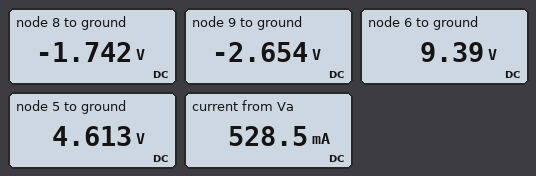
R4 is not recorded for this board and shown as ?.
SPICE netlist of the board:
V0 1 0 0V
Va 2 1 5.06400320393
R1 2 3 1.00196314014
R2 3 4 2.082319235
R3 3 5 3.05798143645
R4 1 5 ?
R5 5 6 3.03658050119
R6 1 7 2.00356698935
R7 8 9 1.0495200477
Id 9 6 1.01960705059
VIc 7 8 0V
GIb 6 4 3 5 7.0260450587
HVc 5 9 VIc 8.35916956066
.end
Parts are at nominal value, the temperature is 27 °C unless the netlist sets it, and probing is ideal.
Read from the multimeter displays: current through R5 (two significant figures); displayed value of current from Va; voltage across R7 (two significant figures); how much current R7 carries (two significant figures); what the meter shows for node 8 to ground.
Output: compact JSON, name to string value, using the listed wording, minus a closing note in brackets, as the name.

{"current through R5": "1.6 A", "displayed value of current from Va": "528.5 mA", "voltage across R7": "910 mV", "how much current R7 carries": "870 mA", "what the meter shows for node 8 to ground": "-1.742 V"}
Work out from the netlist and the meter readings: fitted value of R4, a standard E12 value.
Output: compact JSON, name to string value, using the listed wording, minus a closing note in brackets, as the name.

{"fitted value of R4, a standard E12 value": "3.3 Ω"}
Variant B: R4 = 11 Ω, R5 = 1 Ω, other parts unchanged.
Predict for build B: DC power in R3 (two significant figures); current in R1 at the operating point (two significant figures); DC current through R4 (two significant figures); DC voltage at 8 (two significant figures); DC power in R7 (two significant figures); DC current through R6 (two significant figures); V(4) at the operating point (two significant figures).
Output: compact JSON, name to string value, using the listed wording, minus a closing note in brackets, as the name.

{"DC power in R3": "2.1 mW", "current in R1 at the operating point": "540 mA", "DC current through R4": "500 mA", "DC voltage at 8": "-2.1 V", "DC power in R7": "1.1 W", "DC current through R6": "1.0 A", "V(4) at the operating point": "6.8 V"}
